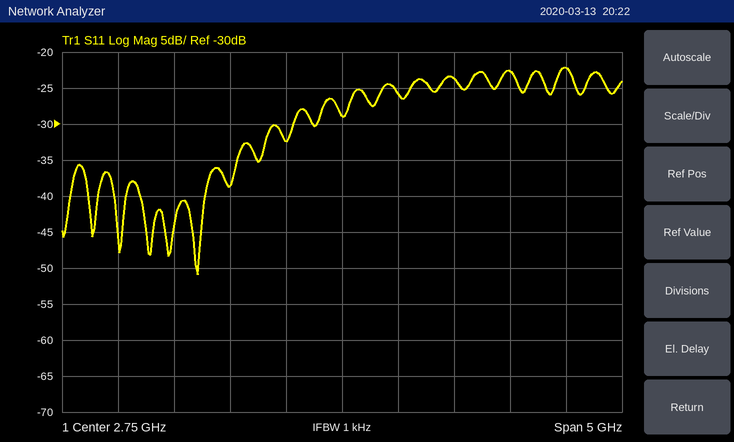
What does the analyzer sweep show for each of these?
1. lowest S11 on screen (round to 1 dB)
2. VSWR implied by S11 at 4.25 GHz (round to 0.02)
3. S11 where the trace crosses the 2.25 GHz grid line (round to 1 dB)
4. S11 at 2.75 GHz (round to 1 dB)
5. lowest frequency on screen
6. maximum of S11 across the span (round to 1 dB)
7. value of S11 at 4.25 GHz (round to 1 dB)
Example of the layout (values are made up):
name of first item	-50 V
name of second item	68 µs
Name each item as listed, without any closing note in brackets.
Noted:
lowest S11 on screen	-51 dB
VSWR implied by S11 at 4.25 GHz	1.16
S11 where the trace crosses the 2.25 GHz grid line	-32 dB
S11 at 2.75 GHz	-29 dB
lowest frequency on screen	250 MHz
maximum of S11 across the span	-22 dB
value of S11 at 4.25 GHz	-23 dB
